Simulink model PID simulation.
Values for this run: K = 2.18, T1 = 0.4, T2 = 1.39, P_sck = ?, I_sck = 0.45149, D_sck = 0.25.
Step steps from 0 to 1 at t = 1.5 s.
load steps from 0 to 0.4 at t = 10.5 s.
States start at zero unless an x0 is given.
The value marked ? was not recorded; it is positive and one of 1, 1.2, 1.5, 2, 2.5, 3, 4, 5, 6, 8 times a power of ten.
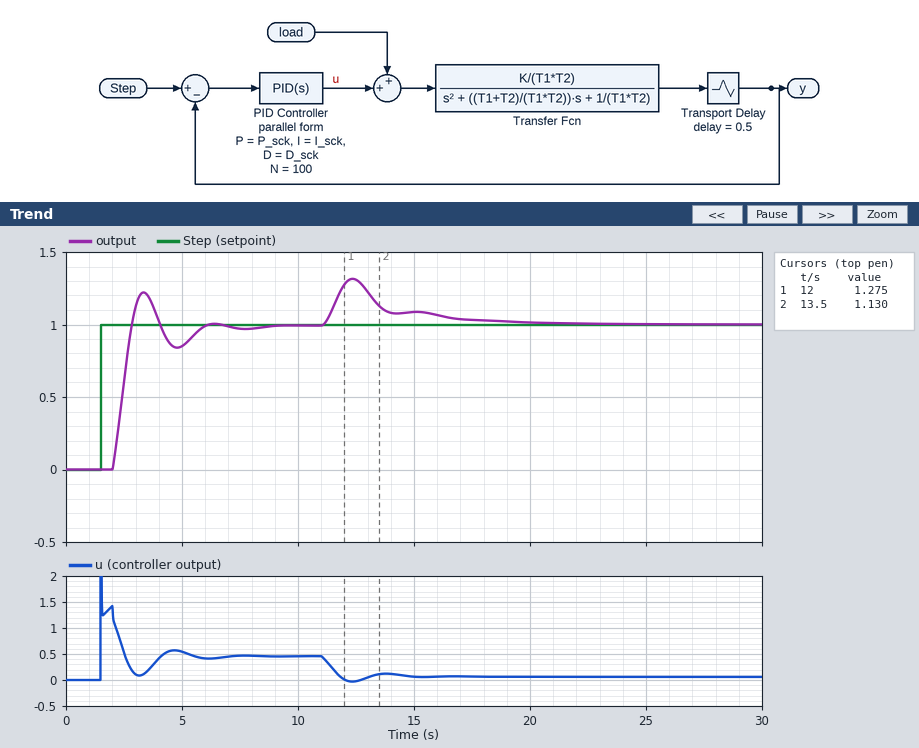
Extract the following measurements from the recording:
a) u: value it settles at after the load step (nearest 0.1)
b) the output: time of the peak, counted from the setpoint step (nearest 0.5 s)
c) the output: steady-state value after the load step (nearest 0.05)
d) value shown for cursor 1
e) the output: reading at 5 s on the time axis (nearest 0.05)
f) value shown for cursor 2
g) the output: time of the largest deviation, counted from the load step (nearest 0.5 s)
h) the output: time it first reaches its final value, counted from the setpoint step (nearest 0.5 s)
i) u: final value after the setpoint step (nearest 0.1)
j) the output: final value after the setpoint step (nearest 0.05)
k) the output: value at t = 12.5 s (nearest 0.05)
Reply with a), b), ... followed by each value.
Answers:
a) 0.1
b) 2.0 s
c) 1.00
d) 1.275
e) 0.85
f) 1.130
g) 2.0 s
h) 1.5 s
i) 0.5
j) 1.00
k) 1.30
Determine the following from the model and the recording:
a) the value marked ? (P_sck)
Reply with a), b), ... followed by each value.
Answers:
a) 1.2
